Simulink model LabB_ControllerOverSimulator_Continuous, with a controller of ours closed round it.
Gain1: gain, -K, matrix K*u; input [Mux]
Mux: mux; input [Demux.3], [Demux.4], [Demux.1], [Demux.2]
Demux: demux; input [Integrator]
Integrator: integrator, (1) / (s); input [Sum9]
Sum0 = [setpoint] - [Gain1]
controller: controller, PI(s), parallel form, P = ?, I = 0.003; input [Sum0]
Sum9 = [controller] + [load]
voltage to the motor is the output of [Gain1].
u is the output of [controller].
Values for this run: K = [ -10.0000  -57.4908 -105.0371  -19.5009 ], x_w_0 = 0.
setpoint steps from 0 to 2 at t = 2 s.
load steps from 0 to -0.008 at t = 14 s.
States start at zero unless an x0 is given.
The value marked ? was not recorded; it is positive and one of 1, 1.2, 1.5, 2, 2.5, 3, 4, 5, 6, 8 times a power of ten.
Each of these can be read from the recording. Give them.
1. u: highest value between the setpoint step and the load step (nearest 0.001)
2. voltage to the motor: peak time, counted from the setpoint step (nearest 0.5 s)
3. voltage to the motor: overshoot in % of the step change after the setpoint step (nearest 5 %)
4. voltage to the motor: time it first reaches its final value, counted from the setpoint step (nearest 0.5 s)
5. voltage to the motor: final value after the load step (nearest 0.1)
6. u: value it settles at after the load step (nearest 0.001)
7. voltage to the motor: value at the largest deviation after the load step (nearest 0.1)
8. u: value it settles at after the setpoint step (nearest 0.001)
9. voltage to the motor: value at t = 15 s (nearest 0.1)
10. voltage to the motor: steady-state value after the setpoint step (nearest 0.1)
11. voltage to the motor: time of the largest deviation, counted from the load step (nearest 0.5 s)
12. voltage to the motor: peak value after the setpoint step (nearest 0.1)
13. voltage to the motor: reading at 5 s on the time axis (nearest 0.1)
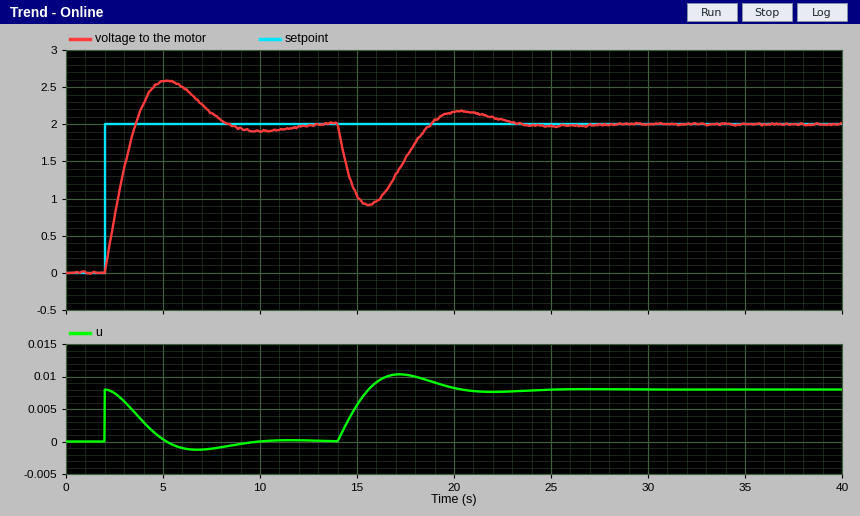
0.008
3.0 s
30 %
1.5 s
2.0
0.008
0.9
0.000
1.0
2.0
1.5 s
2.6
2.6
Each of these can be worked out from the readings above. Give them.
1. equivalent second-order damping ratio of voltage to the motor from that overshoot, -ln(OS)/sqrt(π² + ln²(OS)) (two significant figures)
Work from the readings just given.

0.36
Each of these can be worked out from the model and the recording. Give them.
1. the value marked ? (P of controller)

0.004
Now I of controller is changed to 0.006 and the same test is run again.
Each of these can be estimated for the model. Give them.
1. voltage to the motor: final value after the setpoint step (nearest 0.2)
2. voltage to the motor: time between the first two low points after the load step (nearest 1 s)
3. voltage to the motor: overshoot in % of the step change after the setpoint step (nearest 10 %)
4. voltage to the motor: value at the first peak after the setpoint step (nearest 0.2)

2.0
6 s
40 %
2.8
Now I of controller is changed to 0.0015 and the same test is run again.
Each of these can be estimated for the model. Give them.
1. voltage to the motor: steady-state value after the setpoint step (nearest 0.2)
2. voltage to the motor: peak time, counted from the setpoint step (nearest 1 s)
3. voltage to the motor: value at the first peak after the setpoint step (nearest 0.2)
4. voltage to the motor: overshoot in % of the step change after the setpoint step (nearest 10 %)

2.0
4 s
2.4
20 %
